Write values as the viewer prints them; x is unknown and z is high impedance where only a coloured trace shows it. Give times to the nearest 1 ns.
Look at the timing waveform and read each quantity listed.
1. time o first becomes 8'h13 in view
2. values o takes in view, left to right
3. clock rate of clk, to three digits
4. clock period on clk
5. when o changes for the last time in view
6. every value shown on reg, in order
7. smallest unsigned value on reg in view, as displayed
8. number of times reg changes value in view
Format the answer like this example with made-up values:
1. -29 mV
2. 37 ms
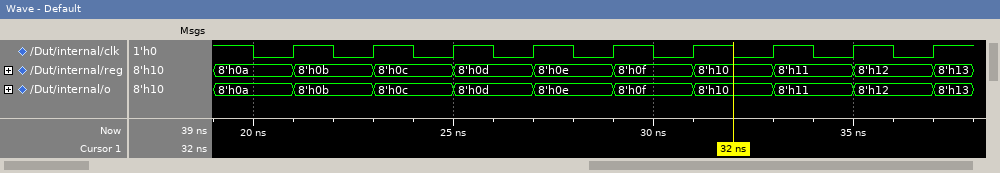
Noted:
1. 37 ns
2. 8'h0a, 8'h0b, 8'h0c, 8'h0d, 8'h0e, 8'h0f, 8'h10, 8'h11, 8'h12, 8'h13
3. 500 MHz
4. 2 ns
5. 37 ns
6. 8'h0a, 8'h0b, 8'h0c, 8'h0d, 8'h0e, 8'h0f, 8'h10, 8'h11, 8'h12, 8'h13
7. 8'h0a
8. 9
